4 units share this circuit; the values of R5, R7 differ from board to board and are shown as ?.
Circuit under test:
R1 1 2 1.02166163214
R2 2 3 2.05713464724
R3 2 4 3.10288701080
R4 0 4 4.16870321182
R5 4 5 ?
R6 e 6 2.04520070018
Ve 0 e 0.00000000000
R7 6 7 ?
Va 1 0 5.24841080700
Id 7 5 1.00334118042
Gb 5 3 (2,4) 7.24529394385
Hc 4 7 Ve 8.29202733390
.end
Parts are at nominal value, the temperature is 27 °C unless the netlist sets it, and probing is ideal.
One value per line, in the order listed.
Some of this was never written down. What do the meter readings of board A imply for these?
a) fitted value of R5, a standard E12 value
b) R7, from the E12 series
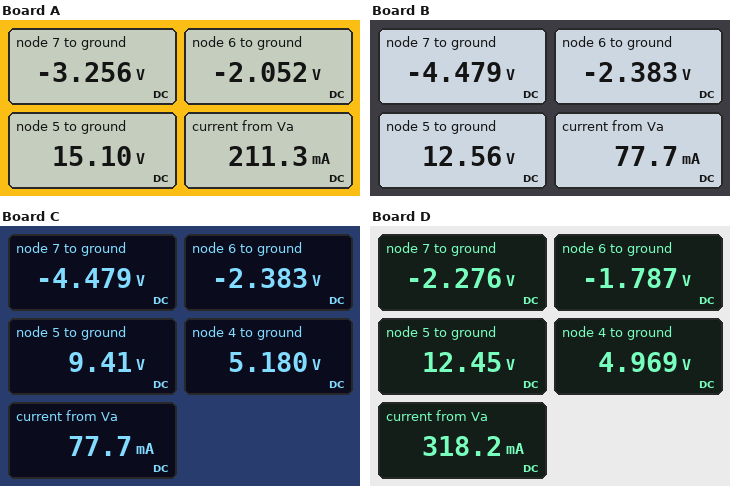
8.2 Ω
1.2 Ω
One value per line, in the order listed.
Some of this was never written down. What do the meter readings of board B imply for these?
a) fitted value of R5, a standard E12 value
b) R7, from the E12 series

6.8 Ω
1.8 Ω
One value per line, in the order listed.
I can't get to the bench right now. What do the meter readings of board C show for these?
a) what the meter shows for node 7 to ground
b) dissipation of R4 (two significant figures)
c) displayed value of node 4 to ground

-4.479 V
6.4 W
5.180 V
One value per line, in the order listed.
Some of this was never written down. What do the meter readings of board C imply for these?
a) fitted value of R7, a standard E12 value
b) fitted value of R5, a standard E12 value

1.8 Ω
3.9 Ω
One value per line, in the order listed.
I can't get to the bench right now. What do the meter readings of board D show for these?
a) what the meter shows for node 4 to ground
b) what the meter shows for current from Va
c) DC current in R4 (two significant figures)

4.969 V
318.2 mA
1.2 A
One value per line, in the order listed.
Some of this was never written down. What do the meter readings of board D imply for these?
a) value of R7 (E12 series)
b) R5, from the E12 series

0.56 Ω
5.6 Ω
